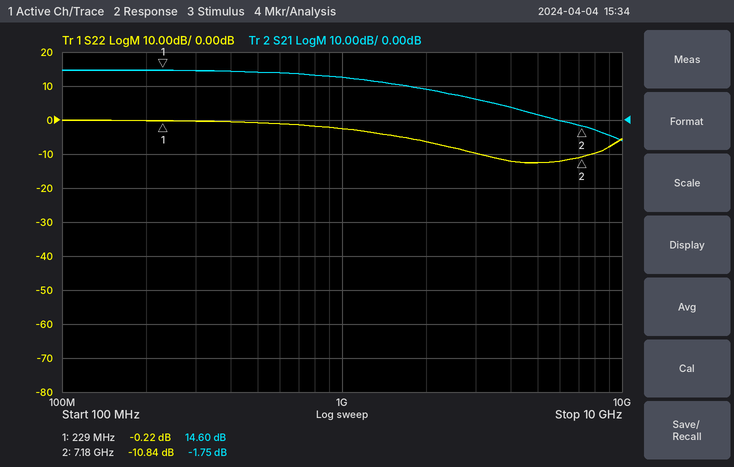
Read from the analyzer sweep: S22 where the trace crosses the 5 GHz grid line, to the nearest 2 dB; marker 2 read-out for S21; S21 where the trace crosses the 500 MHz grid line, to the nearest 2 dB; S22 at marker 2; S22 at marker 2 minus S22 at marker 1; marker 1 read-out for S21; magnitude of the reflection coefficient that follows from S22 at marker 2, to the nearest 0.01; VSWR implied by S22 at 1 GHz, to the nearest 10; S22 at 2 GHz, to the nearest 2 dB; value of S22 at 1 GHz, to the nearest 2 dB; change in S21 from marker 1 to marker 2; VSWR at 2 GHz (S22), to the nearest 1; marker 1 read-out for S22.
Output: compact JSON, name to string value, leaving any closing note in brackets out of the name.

{"S22 where the trace crosses the 5 GHz grid line, to the nearest 2 dB": "-12 dB", "marker 2 read-out for S21": "-1.75 dB", "S21 where the trace crosses the 500 MHz grid line, to the nearest 2 dB": "14 dB", "S22 at marker 2": "-10.84 dB", "S22 at marker 2 minus S22 at marker 1": "-10.62 dB", "marker 1 read-out for S21": "14.60 dB", "magnitude of the reflection coefficient that follows from S22 at marker 2, to the nearest 0.01": "0.29", "VSWR implied by S22 at 1 GHz, to the nearest 10": "10", "S22 at 2 GHz, to the nearest 2 dB": "-6 dB", "value of S22 at 1 GHz, to the nearest 2 dB": "-2 dB", "change in S21 from marker 1 to marker 2": "-16.35 dB", "VSWR at 2 GHz (S22), to the nearest 1": "3", "marker 1 read-out for S22": "-0.22 dB"}
